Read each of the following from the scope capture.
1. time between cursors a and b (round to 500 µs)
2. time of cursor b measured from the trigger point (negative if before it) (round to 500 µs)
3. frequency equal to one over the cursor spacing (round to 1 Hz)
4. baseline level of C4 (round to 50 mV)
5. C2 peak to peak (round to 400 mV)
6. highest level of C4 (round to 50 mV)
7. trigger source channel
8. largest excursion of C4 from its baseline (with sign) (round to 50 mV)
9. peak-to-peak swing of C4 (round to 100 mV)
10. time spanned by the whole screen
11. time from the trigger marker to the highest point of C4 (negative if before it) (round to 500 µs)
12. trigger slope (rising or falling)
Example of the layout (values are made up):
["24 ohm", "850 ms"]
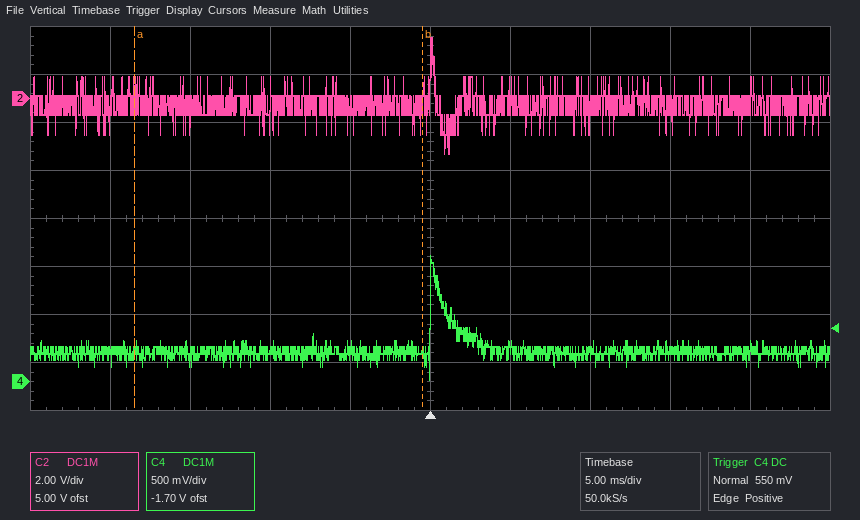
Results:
["18.0 ms", "-500 µs", "56 Hz", "300 mV", "4.8 V", "1.30 V", "C4", "+1.00 V", "1.30 V", "50 ms", "0.0 ms", "rising"]
